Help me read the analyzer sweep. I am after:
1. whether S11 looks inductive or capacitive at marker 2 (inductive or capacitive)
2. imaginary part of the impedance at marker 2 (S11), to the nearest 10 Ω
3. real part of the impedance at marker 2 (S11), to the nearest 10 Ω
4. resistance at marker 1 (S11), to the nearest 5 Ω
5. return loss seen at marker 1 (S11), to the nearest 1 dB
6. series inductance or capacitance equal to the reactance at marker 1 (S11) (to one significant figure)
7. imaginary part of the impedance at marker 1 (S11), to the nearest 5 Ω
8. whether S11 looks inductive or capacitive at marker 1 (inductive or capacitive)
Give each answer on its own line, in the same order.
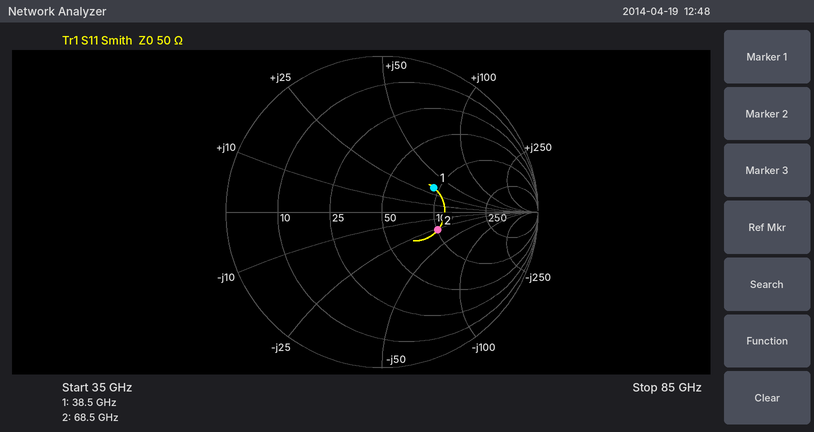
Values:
capacitive
-30 Ω
100 Ω
90 Ω
9 dB
100 pH
+35 Ω
inductive
